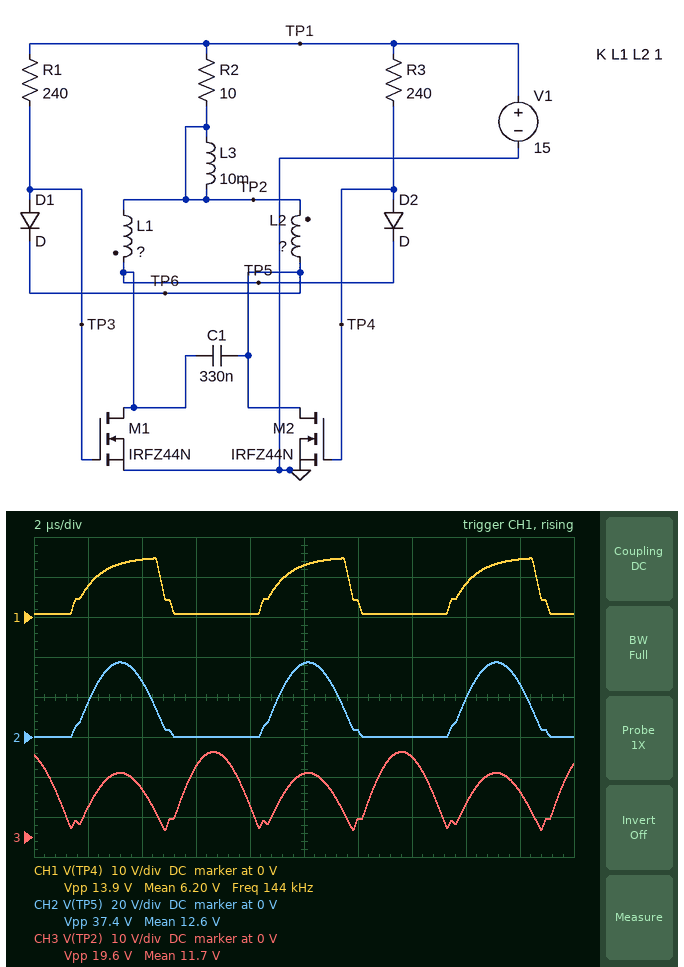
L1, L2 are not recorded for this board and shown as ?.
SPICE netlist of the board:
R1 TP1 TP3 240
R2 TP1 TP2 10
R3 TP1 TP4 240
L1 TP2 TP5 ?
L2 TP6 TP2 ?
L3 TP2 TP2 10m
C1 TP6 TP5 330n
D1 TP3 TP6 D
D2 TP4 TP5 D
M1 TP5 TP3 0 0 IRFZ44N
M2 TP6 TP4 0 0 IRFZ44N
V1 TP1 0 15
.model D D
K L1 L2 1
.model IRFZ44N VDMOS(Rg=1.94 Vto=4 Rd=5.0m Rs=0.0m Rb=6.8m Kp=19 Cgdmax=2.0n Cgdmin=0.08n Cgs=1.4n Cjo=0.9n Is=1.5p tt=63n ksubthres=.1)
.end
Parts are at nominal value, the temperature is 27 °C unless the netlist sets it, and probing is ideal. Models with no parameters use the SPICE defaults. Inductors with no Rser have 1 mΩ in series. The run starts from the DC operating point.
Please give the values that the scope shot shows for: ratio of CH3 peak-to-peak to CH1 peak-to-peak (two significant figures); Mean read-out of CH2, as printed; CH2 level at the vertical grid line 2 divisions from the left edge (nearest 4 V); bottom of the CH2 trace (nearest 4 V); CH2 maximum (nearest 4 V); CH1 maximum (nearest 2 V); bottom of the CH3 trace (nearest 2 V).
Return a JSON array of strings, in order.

["1.4", "12.6 V", "28 V", "0 V", "36 V", "14 V", "2 V"]
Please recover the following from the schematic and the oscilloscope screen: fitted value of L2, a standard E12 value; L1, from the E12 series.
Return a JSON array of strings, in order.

["680 nH", "1.2 µH"]
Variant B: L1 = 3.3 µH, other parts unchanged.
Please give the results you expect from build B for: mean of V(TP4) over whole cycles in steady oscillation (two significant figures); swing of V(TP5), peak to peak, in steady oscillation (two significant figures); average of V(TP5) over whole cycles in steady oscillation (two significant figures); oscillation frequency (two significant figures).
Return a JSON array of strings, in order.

["6.4 V", "34 V", "11 V", "100 kHz"]
